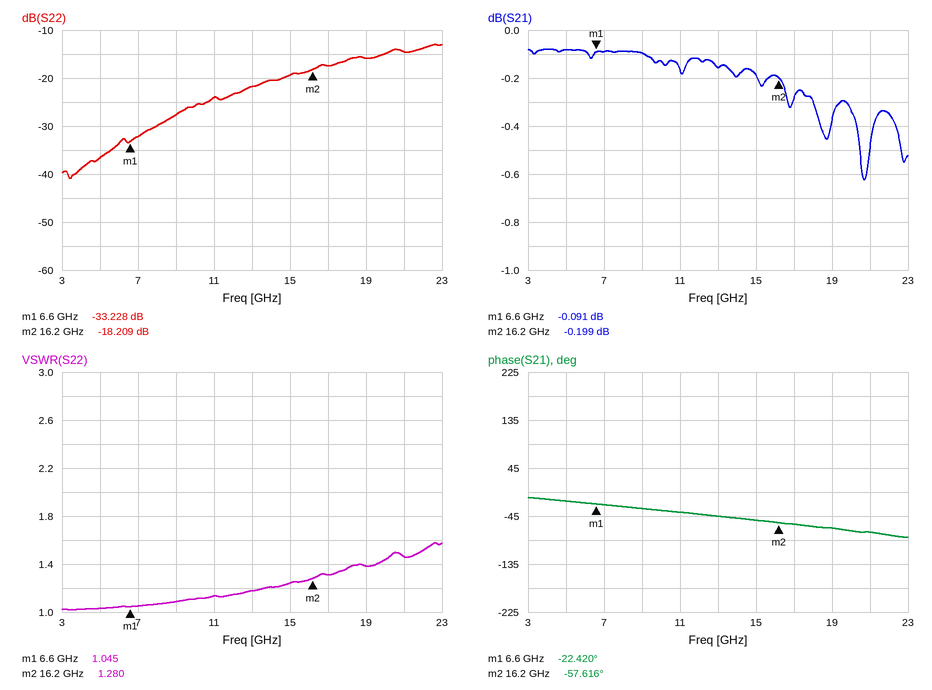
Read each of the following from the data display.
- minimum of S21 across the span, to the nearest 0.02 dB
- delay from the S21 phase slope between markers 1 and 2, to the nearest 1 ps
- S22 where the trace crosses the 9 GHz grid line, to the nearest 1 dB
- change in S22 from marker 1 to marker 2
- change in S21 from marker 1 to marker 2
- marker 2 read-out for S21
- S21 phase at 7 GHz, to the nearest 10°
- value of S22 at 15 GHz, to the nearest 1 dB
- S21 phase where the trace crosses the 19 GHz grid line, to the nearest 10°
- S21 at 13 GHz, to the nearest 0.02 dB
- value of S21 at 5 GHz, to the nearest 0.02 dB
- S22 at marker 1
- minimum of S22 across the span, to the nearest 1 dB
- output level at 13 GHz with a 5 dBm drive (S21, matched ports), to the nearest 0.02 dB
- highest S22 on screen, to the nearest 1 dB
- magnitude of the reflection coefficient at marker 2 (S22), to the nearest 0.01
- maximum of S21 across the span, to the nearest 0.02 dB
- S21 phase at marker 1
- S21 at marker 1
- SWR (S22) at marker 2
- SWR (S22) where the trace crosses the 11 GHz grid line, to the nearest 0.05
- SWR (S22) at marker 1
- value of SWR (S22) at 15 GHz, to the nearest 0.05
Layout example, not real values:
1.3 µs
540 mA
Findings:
-0.62 dB
10 ps
-28 dB
15.019 dB
-0.108 dB
-0.199 dB
-20°
-19 dB
-70°
-0.16 dB
-0.08 dB
-33.228 dB
-41 dB
4.84 dBm
-13 dB
0.12
-0.08 dB
-22.420°
-0.091 dB
1.280
1.15
1.045
1.25
